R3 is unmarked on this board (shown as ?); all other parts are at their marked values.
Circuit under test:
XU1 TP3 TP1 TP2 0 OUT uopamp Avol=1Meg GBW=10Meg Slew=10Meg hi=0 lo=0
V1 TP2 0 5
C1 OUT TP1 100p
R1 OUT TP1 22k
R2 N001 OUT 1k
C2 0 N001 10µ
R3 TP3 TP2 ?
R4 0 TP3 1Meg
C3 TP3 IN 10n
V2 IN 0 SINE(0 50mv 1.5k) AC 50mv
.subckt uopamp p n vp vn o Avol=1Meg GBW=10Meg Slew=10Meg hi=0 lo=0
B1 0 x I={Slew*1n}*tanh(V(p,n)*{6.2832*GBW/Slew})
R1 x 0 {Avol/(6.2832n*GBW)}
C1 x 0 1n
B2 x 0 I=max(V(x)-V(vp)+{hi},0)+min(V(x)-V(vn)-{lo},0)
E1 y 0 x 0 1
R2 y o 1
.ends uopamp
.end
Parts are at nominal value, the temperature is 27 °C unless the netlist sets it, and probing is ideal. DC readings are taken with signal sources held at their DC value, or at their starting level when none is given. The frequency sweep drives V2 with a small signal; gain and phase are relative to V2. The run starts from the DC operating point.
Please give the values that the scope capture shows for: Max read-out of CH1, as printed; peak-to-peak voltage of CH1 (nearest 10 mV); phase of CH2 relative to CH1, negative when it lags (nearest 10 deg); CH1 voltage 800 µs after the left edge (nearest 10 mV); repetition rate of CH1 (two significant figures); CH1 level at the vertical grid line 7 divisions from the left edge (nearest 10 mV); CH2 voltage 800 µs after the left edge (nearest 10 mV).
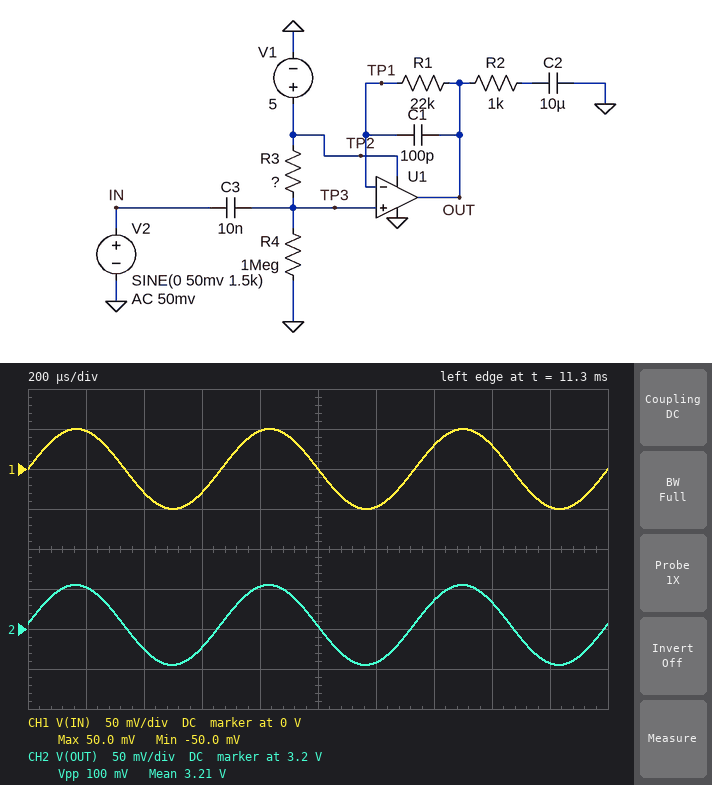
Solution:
50.0 mV
100 mV
0 deg
50 mV
1.5 kHz
30 mV
3.25 V
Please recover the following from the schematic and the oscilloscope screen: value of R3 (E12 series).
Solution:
560 kΩ
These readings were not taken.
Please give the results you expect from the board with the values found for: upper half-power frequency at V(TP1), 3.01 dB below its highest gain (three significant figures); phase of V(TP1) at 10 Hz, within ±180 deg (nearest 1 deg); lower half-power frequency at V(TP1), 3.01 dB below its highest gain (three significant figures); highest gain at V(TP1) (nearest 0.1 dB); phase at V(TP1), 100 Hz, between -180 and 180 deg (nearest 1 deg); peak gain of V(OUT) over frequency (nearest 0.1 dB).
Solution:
9.99 MHz
77 deg
44.3 Hz
0 dB
24 deg
0 dB
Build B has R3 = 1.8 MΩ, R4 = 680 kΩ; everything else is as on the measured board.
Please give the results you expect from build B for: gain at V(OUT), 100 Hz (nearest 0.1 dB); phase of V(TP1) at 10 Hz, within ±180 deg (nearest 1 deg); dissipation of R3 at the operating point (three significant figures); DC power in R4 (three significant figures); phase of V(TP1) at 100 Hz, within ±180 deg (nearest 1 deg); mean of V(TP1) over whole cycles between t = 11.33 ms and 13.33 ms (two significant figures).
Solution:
-0.4 dB
73 deg
7.32 µW
2.76 µW
18 deg
1.4 V
